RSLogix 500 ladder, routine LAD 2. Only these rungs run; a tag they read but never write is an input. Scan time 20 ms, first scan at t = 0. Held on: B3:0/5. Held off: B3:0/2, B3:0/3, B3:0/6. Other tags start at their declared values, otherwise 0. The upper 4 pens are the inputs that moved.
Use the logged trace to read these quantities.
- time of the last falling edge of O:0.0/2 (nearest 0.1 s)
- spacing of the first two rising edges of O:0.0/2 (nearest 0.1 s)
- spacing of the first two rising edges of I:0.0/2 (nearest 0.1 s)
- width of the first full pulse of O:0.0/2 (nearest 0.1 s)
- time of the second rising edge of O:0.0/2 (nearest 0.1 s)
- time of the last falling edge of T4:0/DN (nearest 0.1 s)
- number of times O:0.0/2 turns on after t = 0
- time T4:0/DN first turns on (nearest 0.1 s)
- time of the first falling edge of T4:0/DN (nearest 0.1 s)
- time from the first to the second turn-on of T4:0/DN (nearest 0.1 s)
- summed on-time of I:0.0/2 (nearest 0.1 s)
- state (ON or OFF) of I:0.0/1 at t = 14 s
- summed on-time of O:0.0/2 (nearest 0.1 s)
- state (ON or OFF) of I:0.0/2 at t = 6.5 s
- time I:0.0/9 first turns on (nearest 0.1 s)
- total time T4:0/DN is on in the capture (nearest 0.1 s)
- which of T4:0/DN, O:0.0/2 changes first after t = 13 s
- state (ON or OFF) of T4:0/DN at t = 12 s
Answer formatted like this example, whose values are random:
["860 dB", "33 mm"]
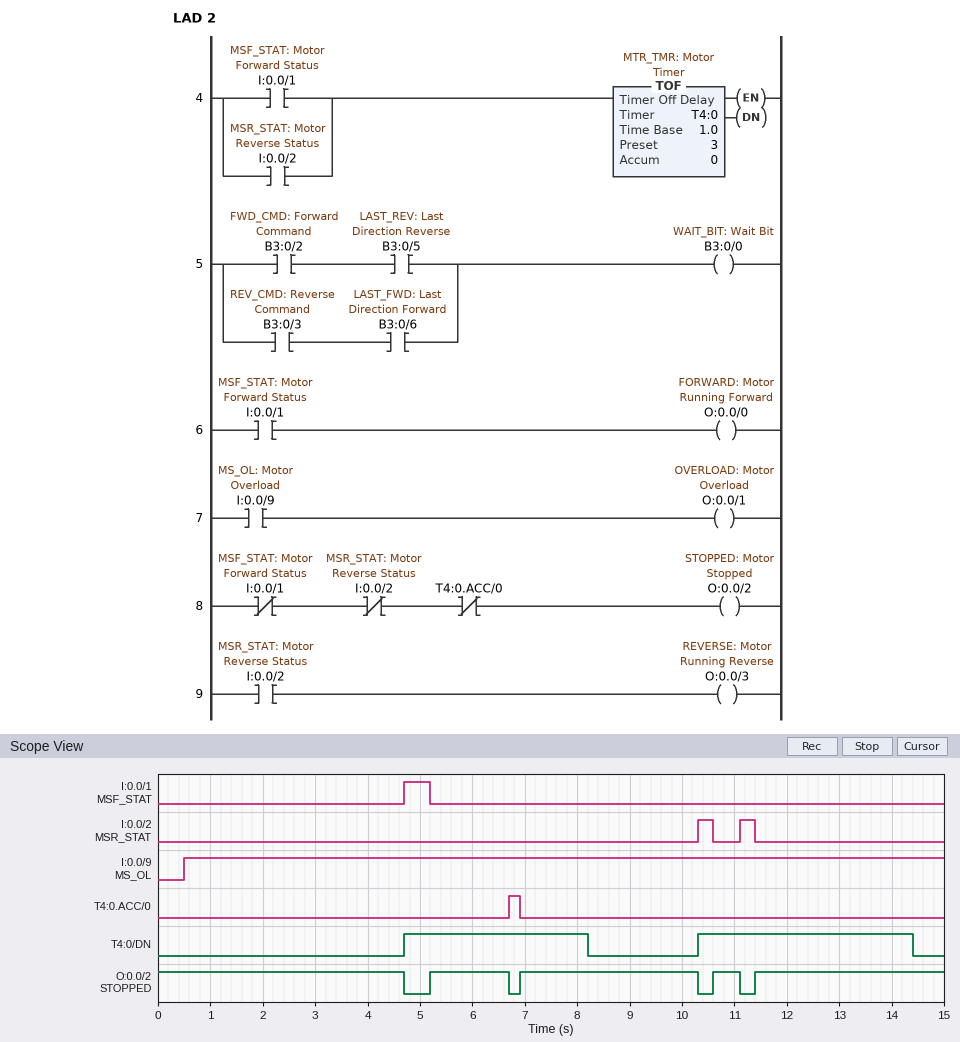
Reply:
["11.1 s", "1.7 s", "0.8 s", "1.5 s", "6.9 s", "14.4 s", "4", "4.7 s", "8.2 s", "5.6 s", "0.6 s", "OFF", "13.7 s", "OFF", "0.5 s", "7.6 s", "T4:0/DN", "ON"]
